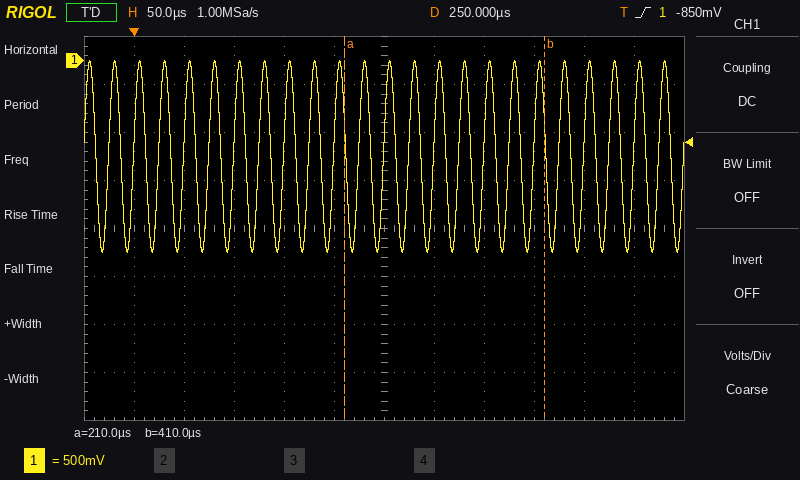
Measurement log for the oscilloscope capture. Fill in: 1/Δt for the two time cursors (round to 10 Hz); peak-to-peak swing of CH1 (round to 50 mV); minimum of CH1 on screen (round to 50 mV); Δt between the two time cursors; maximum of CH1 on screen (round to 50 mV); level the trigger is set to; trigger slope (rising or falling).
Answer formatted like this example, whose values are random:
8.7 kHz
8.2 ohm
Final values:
5.00 kHz
2.00 V
-2.00 V
200 µs
0 mV
-850 mV
rising
